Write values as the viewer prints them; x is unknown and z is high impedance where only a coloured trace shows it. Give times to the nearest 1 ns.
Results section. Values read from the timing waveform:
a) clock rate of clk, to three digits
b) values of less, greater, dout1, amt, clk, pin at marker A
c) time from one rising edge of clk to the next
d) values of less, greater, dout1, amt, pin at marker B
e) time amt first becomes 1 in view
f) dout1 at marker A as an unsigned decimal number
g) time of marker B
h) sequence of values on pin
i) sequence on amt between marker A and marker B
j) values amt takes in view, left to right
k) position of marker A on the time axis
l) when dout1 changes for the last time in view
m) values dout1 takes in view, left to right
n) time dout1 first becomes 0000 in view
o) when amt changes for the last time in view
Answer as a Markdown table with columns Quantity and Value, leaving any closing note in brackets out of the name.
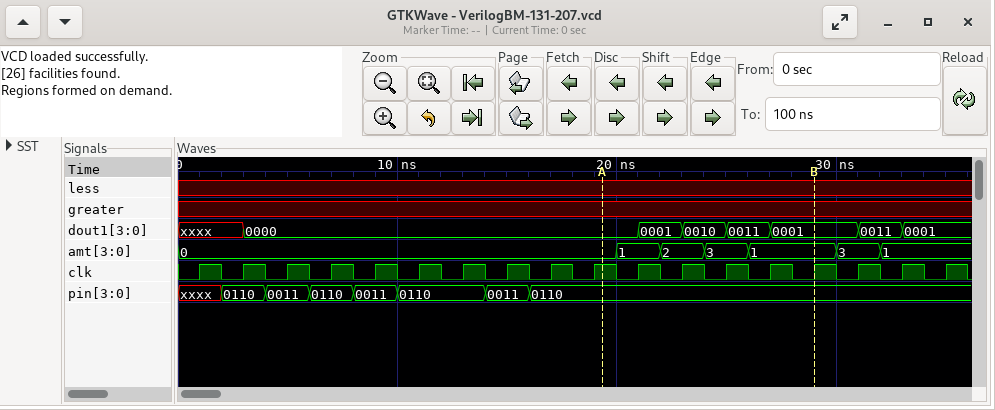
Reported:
| Quantity | Value |
|---|---|
| clock rate of clk, to three digits | 500 MHz |
| values of less, greater, dout1, amt, clk, pin at marker A | less=x, greater=x, dout1=0000, amt=0, clk=1, pin=0110 |
| time from one rising edge of clk to the next | 2 ns |
| values of less, greater, dout1, amt, pin at marker B | less=x, greater=x, dout1=0001, amt=1, pin=0110 |
| time amt first becomes 1 in view | 20 ns |
| dout1 at marker A as an unsigned decimal number | 0 |
| time of marker B | 29 ns |
| sequence of values on pin | xxxx, 0110, 0011, 0110, 0011, 0110, 0011, 0110 |
| sequence on amt between marker A and marker B | 0, 1, 2, 3, 1 |
| values amt takes in view, left to right | 0, 1, 2, 3, 1, 3, 1 |
| position of marker A on the time axis | 19 ns |
| when dout1 changes for the last time in view | 33 ns |
| values dout1 takes in view, left to right | xxxx, 0000, 0001, 0010, 0011, 0001, 0011, 0001 |
| time dout1 first becomes 0000 in view | 3 ns |
| when amt changes for the last time in view | 32 ns |
